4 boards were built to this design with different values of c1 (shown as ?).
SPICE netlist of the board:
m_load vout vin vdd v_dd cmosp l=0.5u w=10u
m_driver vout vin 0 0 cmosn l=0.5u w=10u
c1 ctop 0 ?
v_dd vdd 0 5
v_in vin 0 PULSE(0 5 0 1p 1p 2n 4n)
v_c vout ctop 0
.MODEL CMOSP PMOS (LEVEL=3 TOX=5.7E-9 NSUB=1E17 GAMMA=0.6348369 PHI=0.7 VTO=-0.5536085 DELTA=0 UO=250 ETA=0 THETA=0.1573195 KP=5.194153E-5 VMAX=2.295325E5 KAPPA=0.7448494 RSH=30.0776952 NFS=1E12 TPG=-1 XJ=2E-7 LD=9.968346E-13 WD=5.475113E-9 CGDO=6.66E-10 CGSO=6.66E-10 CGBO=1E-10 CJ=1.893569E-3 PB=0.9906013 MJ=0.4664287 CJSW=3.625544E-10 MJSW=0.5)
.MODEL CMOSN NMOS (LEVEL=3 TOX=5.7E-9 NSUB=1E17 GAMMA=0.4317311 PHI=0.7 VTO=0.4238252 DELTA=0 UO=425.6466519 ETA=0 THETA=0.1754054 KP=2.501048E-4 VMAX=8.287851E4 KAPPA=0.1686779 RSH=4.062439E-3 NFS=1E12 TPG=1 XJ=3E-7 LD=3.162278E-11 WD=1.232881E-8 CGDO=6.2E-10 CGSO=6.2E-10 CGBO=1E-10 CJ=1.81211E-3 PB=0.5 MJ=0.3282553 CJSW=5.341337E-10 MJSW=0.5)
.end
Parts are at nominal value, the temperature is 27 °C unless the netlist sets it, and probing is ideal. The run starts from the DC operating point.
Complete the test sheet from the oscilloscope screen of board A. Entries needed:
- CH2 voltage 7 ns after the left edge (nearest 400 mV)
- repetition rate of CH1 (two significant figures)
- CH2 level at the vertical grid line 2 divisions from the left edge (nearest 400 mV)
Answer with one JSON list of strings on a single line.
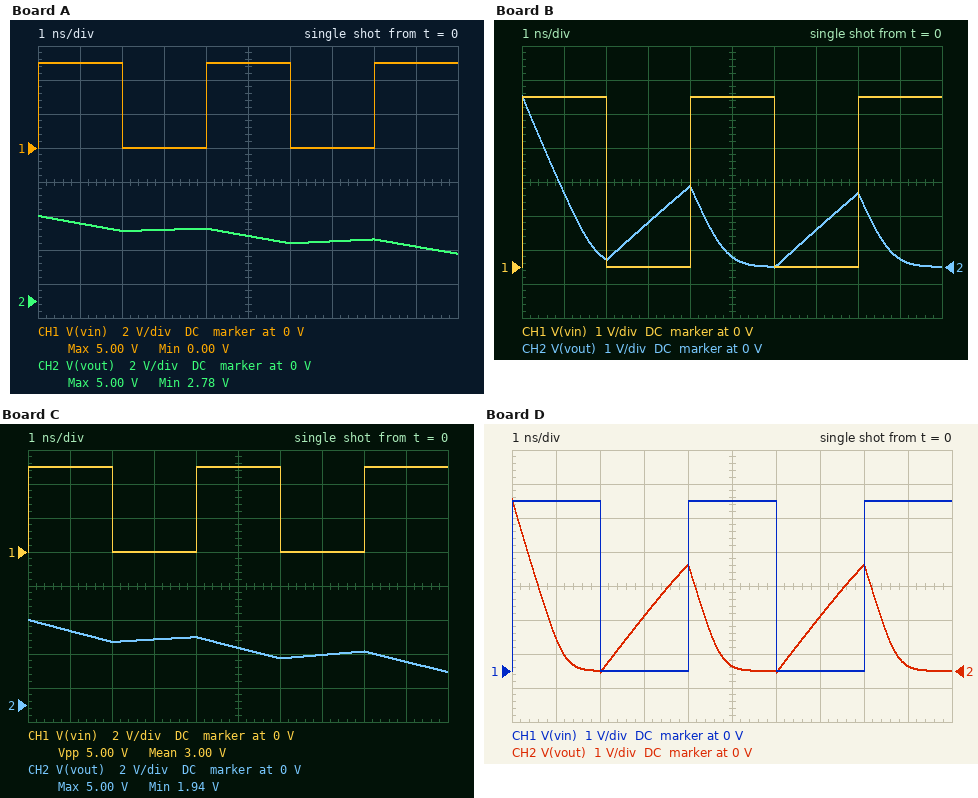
["3.6 V", "250 MHz", "4.0 V"]
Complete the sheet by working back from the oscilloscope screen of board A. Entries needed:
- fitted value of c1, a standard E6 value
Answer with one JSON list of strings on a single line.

["22 pF"]
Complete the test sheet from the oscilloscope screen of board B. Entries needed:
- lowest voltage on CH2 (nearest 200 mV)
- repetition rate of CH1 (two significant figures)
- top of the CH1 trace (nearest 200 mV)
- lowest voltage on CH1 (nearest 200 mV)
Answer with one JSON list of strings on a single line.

["0 V", "250 MHz", "5.0 V", "0 V"]
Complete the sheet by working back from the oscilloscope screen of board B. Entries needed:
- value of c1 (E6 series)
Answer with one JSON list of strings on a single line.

["3.3 pF"]
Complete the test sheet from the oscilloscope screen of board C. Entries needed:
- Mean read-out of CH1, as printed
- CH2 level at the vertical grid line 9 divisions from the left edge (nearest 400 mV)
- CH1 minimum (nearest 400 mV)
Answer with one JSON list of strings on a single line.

["3.00 V", "2.4 V", "0 V"]
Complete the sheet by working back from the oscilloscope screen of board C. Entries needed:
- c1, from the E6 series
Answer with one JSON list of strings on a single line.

["15 pF"]
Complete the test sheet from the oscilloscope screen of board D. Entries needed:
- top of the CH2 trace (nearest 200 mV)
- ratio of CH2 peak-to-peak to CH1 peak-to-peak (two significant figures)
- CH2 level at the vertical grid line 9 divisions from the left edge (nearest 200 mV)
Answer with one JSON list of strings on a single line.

["5.0 V", "1.0", "200 mV"]
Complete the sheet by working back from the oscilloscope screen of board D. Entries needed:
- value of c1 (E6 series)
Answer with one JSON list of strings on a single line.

["2.2 pF"]
